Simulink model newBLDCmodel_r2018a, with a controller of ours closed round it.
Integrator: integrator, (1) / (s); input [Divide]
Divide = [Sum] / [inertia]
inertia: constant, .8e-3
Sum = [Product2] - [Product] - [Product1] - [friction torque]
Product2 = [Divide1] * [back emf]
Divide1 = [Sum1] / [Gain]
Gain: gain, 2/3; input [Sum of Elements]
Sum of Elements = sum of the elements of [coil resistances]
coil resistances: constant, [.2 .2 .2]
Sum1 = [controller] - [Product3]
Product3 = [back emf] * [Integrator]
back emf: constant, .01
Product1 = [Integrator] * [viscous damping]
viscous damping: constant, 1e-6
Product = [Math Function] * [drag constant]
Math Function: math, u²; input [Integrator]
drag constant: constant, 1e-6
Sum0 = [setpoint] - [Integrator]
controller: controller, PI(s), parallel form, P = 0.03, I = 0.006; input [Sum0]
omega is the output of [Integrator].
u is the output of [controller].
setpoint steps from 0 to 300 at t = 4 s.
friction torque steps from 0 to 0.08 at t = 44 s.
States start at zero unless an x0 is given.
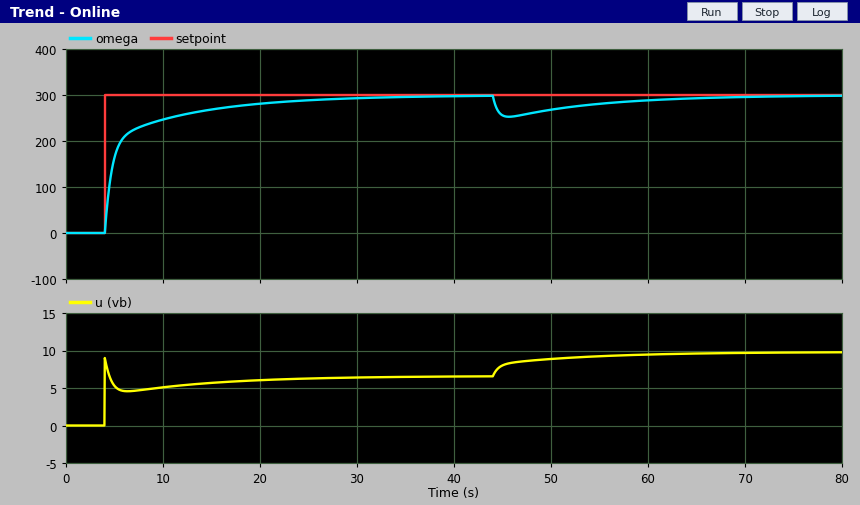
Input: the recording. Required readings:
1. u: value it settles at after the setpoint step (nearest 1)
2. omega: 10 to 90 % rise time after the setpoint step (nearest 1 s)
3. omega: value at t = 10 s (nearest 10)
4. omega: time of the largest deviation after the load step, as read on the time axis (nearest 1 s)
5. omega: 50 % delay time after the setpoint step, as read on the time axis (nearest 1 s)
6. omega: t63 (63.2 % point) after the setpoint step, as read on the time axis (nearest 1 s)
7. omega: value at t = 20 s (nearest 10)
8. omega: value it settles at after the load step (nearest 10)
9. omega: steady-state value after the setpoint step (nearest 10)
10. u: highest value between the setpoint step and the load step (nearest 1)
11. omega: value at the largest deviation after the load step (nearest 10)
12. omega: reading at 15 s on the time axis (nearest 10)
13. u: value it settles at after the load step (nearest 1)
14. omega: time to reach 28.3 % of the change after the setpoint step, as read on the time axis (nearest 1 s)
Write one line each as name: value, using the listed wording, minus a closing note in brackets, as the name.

u: value it settles at after the setpoint step: 7
omega: 10 to 90 % rise time after the setpoint step: 11 s
omega: value at t = 10 s: 250
omega: time of the largest deviation after the load step, as read on the time axis: 46 s
omega: 50 % delay time after the setpoint step, as read on the time axis: 5 s
omega: t63 (63.2 % point) after the setpoint step, as read on the time axis: 5 s
omega: value at t = 20 s: 280
omega: value it settles at after the load step: 300
omega: steady-state value after the setpoint step: 300
u: highest value between the setpoint step and the load step: 9
omega: value at the largest deviation after the load step: 250
omega: reading at 15 s on the time axis: 270
u: value it settles at after the load step: 10
omega: time to reach 28.3 % of the change after the setpoint step, as read on the time axis: 4 s
